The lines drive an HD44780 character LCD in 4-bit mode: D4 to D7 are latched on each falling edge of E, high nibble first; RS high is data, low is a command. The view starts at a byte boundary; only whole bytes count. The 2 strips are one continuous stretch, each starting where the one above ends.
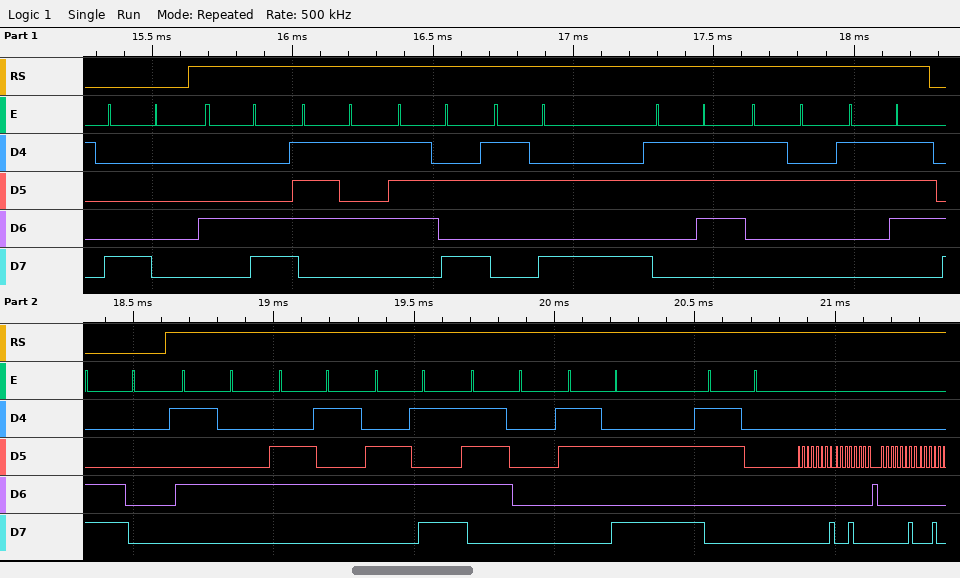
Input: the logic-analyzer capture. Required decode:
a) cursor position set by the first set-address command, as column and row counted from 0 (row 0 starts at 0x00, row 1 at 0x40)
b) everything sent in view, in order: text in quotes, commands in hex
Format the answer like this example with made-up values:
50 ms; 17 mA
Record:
column 0, row 0; 0x80 "Luz:727" 0xC0 "Temp:0"
